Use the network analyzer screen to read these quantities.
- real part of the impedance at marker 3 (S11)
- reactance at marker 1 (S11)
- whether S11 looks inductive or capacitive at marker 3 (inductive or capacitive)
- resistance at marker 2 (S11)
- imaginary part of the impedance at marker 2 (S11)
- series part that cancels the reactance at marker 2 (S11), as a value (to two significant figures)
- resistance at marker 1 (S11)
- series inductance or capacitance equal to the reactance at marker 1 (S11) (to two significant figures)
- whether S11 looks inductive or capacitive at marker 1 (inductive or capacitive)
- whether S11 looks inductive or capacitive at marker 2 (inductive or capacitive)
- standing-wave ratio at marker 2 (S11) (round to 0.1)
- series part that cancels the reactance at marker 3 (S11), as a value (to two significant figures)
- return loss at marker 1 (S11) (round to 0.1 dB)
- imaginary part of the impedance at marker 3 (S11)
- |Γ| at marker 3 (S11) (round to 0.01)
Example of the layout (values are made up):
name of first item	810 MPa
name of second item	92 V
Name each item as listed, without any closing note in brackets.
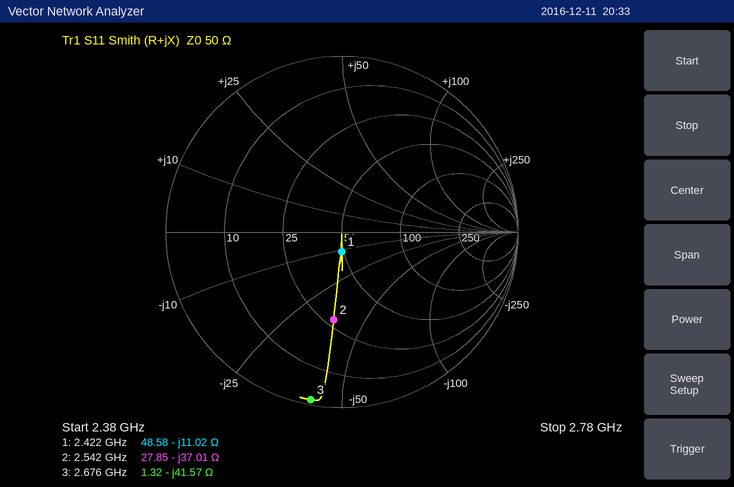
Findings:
real part of the impedance at marker 3	1.32 Ω
reactance at marker 1	-11.02 Ω
whether S11 looks inductive or capacitive at marker 3	capacitive
resistance at marker 2	27.85 Ω
imaginary part of the impedance at marker 2	-37.01 Ω
series part that cancels the reactance at marker 2 (S11), as a value	2.3 nH
resistance at marker 1	48.58 Ω
series inductance or capacitance equal to the reactance at marker 1 (S11)	6.0 pF
whether S11 looks inductive or capacitive at marker 1	capacitive
whether S11 looks inductive or capacitive at marker 2	capacitive
standing-wave ratio at marker 2 (S11)	3.0
series part that cancels the reactance at marker 3 (S11), as a value	2.5 nH
return loss at marker 1 (S11)	19.0 dB
imaginary part of the impedance at marker 3	-41.57 Ω
|Γ| at marker 3 (S11)	0.97
